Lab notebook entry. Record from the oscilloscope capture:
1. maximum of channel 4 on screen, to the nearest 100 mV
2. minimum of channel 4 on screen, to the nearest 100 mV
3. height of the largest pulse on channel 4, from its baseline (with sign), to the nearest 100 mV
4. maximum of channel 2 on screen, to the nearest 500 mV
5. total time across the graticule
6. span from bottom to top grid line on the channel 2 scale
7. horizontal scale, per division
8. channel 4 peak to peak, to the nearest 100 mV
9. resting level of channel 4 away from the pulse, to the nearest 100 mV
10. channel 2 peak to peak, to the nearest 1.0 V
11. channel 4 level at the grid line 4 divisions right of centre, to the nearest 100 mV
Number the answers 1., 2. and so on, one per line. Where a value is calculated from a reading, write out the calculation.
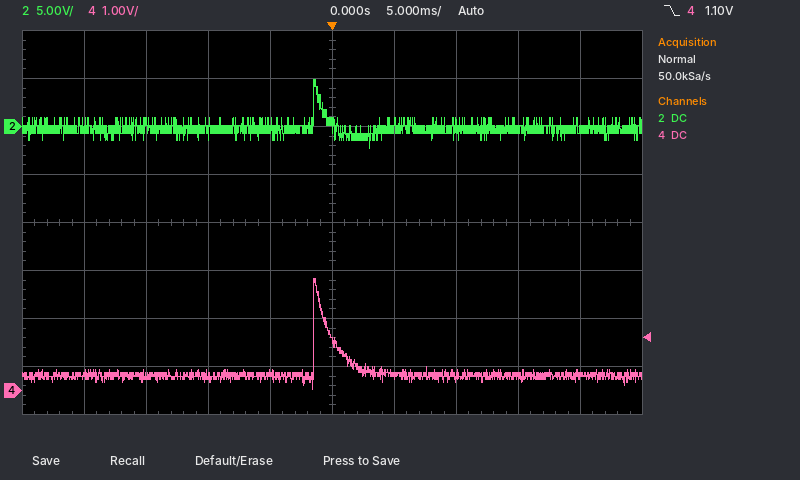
1. 2.3 V
2. 0.0 V
3. 2.3 V − (300 mV) = +2.0 V
4. 5.0 V
5. 50 ms
6. 40 V
7. 5 ms
8. 2.3 V − (0.0 V) = 2.3 V
9. 300 mV
10. 7.0 V
11. 300 mV
